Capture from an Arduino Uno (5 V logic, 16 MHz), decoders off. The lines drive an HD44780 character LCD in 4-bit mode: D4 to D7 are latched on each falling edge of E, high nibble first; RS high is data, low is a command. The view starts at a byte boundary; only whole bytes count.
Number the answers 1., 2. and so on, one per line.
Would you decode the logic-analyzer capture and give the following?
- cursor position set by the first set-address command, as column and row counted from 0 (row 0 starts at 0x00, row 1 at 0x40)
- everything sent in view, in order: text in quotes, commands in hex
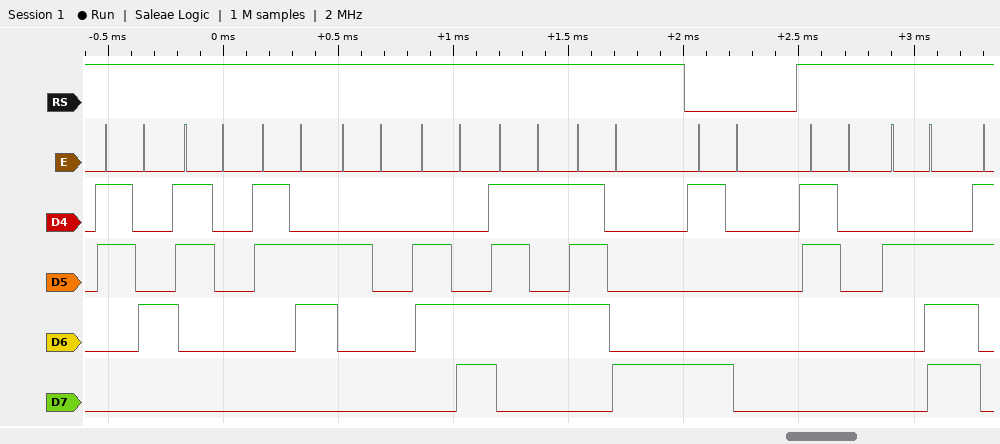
1. column 16, row 0
2. "406 lux" 0x90 "0."
